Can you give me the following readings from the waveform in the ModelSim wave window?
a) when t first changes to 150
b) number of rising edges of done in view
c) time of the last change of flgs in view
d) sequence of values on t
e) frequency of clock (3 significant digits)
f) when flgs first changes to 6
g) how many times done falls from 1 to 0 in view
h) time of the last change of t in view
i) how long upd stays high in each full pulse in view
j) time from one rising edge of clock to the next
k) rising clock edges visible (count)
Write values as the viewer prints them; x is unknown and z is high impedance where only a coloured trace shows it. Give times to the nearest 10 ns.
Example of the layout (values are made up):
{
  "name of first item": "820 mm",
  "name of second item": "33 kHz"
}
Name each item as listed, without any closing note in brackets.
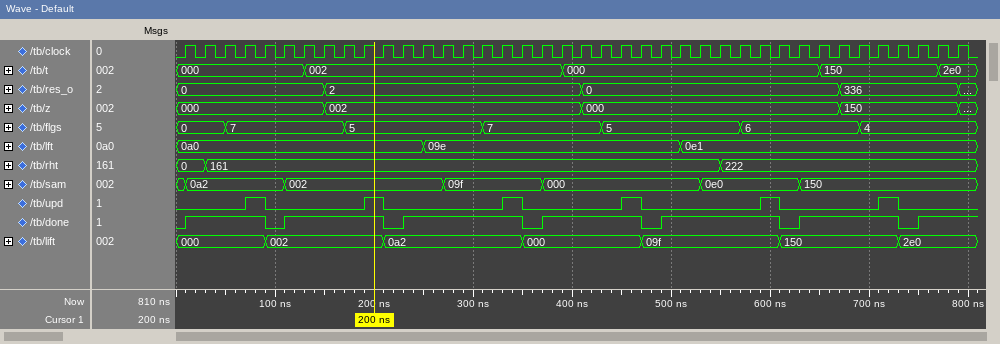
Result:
{
  "when t first changes to 150": "650 ns",
  "number of rising edges of done in view": "7",
  "time of the last change of flgs in view": "690 ns",
  "sequence of values on t": "000, 002, 000, 150, 2e0",
  "frequency of clock": "50.0 MHz",
  "when flgs first changes to 6": "570 ns",
  "how many times done falls from 1 to 0 in view": "6",
  "time of the last change of t in view": "770 ns",
  "how long upd stays high in each full pulse in view": "20 ns, 20 ns, 20 ns, 20 ns, 20 ns, 20 ns",
  "time from one rising edge of clock to the next": "20 ns",
  "rising clock edges visible": "40"
}
